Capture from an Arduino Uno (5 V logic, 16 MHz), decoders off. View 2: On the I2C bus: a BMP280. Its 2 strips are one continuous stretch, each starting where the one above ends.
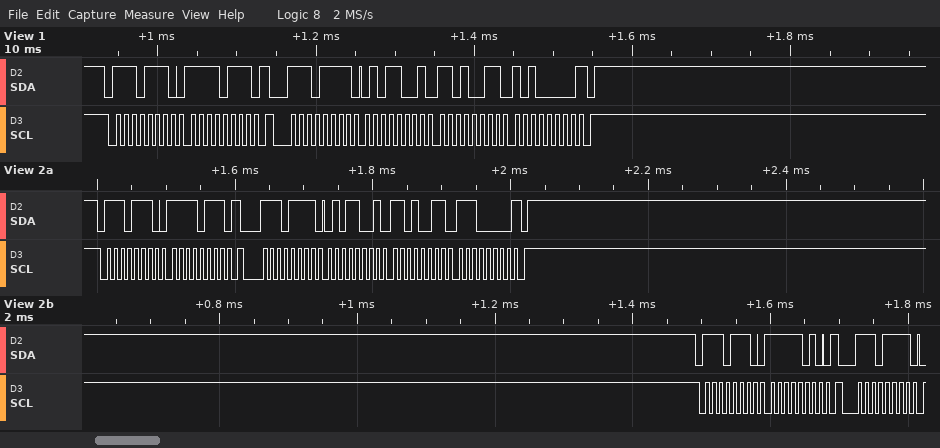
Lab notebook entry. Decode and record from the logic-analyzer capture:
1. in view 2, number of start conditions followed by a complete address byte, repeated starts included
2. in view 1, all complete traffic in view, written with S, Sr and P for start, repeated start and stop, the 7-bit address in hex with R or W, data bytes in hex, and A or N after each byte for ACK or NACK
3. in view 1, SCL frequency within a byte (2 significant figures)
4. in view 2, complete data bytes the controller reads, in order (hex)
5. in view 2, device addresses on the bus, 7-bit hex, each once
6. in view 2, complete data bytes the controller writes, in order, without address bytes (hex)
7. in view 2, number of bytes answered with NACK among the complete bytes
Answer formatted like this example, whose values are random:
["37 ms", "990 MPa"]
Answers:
["4", "S 77W A F7 A Sr 77R A 59 A D3 A A0 N P", "100 kHz", "59 D3 E0", "0x77", "F7 FA", "1"]
